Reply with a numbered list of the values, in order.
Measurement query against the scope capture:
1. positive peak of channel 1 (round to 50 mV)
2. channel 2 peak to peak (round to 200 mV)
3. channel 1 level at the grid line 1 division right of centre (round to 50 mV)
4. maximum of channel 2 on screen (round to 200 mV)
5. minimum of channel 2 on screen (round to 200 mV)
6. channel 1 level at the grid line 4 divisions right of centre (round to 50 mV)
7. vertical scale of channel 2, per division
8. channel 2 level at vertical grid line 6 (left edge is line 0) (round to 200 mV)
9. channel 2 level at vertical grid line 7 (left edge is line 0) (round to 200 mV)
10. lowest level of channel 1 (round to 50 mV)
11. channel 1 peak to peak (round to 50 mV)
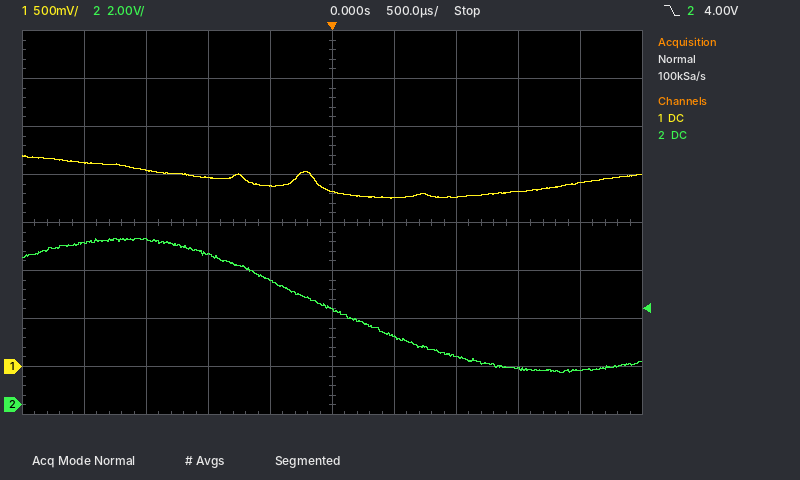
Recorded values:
1. 2.20 V
2. 5.6 V
3. 1.75 V
4. 7.0 V
5. 1.4 V
6. 1.90 V
7. 2 V
8. 2.8 V
9. 2.0 V
10. 1.75 V
11. 450 mV
